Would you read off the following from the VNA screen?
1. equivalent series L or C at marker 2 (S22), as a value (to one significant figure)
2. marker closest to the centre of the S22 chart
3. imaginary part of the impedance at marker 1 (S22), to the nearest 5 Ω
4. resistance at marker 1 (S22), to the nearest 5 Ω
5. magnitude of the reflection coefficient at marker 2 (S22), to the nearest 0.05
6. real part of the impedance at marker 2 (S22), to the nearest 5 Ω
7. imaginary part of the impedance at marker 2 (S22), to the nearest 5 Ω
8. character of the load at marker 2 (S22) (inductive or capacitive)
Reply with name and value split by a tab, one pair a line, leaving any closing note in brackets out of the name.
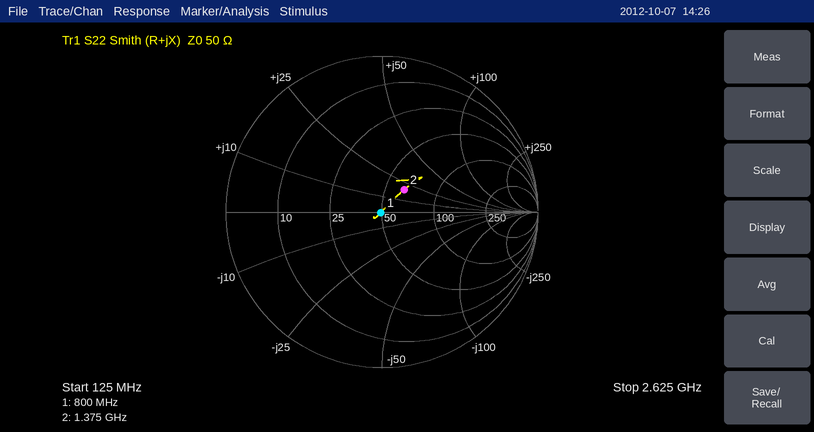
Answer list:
equivalent series L or C at marker 2 (S22), as a value	2 nH
marker closest to the centre of the S22 chart	marker 1
imaginary part of the impedance at marker 1 (S22), to the nearest 5 Ω	0 Ω
resistance at marker 1 (S22), to the nearest 5 Ω	50 Ω
magnitude of the reflection coefficient at marker 2 (S22), to the nearest 0.05	0.20
real part of the impedance at marker 2 (S22), to the nearest 5 Ω	65 Ω
imaginary part of the impedance at marker 2 (S22), to the nearest 5 Ω	+20 Ω
character of the load at marker 2 (S22)	inductive
